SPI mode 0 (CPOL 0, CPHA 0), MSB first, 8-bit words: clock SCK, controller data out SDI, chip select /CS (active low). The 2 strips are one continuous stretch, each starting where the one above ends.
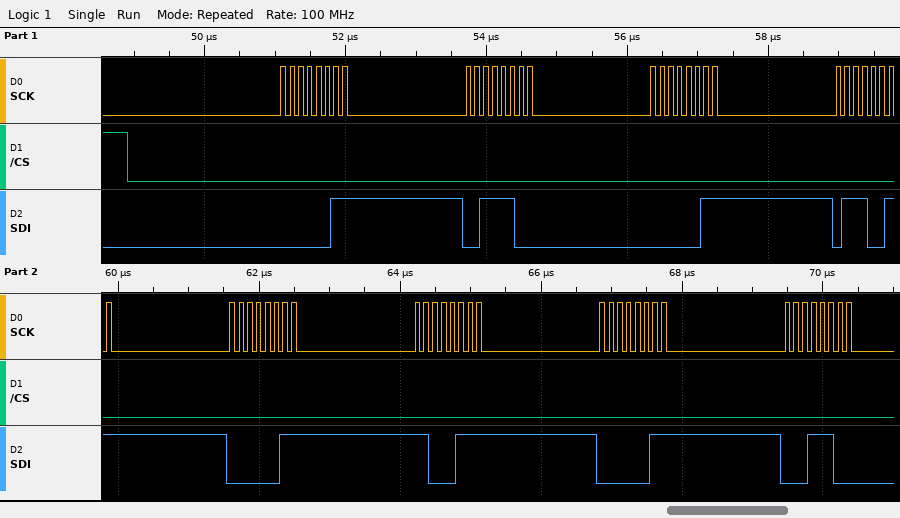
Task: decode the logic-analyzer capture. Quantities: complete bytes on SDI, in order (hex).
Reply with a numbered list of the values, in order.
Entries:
1. 03 3C 03 73 03 C7 03 1C
